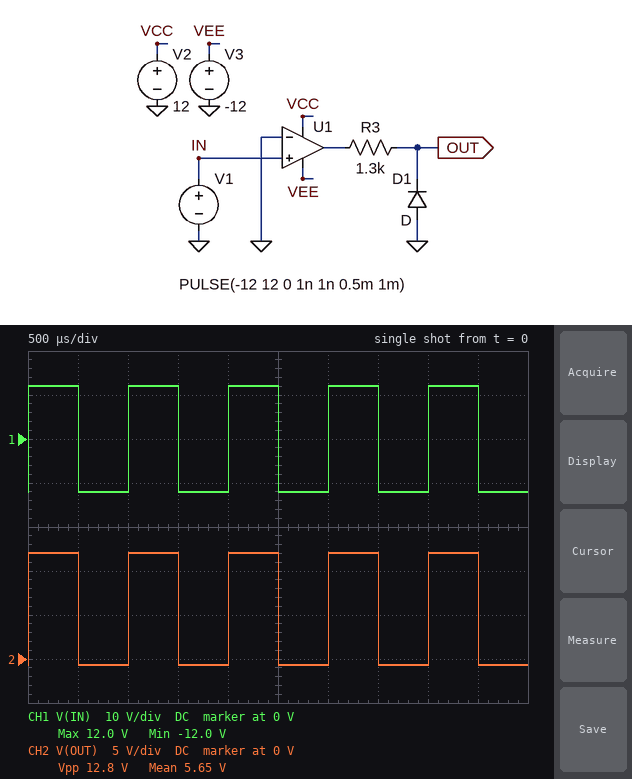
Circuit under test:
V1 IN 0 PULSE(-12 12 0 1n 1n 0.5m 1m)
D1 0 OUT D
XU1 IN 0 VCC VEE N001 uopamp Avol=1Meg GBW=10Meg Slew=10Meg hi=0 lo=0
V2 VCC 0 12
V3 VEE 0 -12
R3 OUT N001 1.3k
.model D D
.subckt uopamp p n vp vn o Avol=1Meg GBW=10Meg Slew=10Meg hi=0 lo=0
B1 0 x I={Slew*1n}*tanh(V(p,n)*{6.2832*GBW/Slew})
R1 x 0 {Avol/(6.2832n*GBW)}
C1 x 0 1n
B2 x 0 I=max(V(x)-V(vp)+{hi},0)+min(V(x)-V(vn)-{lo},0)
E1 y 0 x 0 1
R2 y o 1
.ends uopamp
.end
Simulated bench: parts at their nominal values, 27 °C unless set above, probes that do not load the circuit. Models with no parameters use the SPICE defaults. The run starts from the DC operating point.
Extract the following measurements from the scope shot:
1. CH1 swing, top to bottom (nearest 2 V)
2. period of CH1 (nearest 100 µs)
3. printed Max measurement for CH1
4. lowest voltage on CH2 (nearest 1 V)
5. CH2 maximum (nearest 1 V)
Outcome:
24 V
1.0 ms
12.0 V
-1 V
12 V
